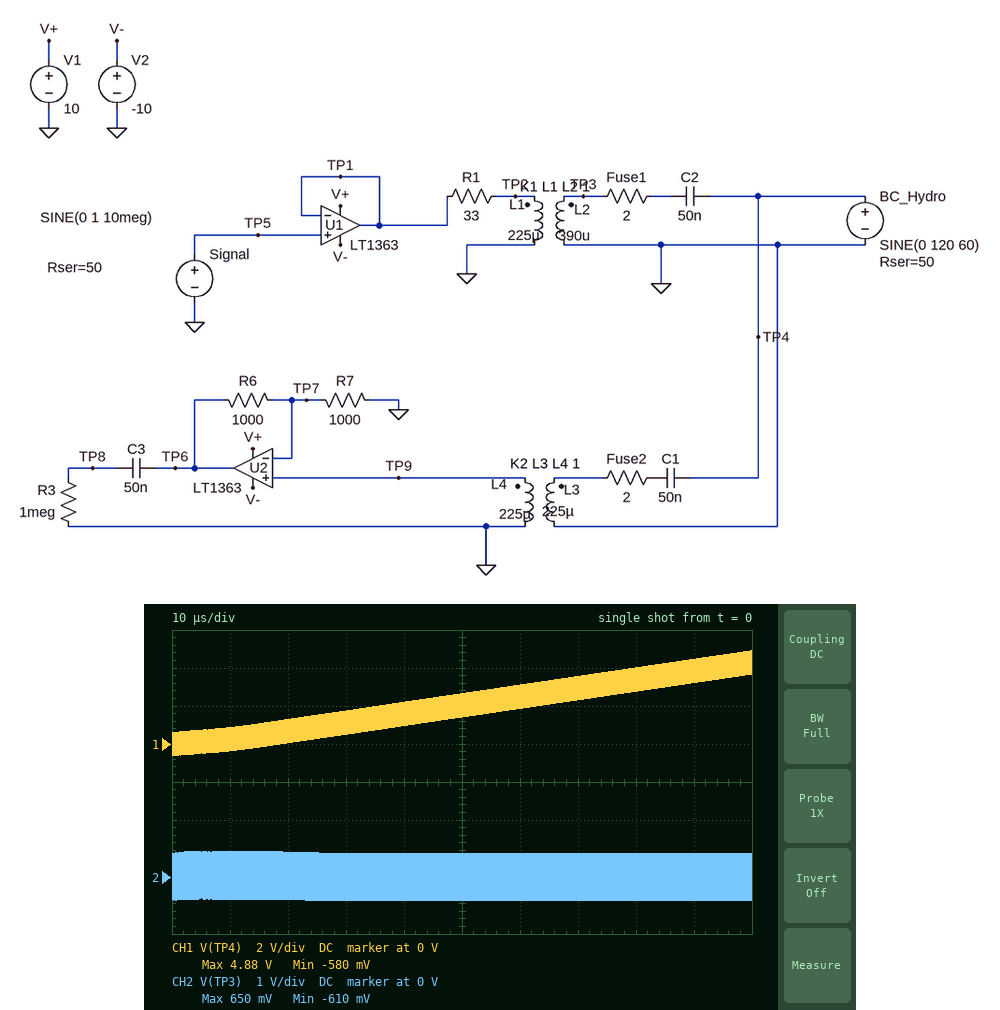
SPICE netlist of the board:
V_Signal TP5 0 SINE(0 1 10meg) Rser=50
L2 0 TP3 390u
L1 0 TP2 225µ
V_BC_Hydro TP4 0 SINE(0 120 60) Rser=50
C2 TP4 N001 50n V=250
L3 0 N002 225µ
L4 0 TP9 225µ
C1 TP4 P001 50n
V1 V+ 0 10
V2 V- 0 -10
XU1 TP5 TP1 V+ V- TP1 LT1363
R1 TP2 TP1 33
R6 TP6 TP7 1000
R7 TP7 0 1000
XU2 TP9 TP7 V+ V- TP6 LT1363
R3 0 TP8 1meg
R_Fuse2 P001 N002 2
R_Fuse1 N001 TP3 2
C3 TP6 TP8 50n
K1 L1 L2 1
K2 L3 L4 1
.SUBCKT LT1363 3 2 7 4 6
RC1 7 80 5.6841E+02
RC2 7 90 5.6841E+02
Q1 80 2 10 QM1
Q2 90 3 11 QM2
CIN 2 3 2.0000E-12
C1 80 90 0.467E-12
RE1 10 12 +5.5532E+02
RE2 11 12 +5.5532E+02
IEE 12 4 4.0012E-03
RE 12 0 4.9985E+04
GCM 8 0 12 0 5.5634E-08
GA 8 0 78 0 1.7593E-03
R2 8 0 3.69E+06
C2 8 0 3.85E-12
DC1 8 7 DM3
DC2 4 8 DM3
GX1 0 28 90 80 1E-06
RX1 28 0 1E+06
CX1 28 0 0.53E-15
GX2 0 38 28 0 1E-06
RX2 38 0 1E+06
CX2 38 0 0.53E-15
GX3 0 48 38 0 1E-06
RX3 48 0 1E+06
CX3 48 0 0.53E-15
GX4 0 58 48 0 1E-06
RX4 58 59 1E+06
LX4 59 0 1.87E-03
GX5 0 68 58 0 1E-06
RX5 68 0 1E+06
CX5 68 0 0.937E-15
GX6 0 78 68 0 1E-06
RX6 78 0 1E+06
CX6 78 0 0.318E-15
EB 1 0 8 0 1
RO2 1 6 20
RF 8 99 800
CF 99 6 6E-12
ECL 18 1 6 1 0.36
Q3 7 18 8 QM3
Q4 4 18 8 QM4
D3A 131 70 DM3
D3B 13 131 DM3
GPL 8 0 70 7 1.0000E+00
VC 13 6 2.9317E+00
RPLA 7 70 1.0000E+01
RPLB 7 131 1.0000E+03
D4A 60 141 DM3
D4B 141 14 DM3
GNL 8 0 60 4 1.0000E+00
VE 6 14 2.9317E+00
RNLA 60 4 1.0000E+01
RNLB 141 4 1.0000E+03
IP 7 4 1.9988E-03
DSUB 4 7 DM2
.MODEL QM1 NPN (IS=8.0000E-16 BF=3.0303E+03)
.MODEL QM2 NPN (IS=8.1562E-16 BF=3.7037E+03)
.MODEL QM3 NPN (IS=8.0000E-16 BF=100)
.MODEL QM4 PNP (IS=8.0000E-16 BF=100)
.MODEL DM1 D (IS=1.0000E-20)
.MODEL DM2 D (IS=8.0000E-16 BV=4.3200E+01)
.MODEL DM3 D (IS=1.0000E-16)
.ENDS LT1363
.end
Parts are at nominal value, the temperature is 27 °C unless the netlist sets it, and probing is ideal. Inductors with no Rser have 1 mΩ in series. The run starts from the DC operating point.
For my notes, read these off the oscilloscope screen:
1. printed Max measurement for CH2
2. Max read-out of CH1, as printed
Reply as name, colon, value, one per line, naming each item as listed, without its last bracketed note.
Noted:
printed Max measurement for CH2: 650 mV
Max read-out of CH1, as printed: 4.88 V
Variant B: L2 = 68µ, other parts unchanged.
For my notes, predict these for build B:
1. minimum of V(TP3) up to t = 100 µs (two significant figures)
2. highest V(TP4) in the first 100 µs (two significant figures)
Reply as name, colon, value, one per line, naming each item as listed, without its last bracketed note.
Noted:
minimum of V(TP3) up to t = 100 µs: -460 mV
highest V(TP4) in the first 100 µs: 4.7 V
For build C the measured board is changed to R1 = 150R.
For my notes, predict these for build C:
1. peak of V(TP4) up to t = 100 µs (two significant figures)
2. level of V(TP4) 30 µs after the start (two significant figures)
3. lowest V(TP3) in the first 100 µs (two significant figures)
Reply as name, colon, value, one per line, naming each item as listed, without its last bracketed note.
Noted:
peak of V(TP4) up to t = 100 µs: 4.5 V
level of V(TP4) 30 µs after the start: 1.1 V
lowest V(TP3) in the first 100 µs: -240 mV
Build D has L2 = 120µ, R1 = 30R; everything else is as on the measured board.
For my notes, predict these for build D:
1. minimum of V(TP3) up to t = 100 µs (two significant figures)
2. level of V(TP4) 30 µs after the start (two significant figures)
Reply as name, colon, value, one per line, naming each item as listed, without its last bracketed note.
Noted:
minimum of V(TP3) up to t = 100 µs: -550 mV
level of V(TP4) 30 µs after the start: 1.0 V
